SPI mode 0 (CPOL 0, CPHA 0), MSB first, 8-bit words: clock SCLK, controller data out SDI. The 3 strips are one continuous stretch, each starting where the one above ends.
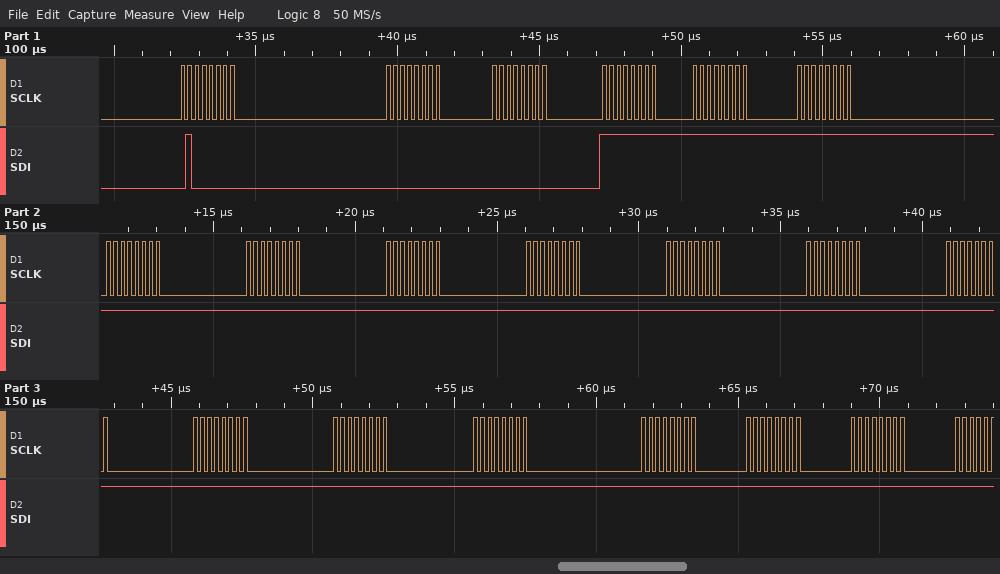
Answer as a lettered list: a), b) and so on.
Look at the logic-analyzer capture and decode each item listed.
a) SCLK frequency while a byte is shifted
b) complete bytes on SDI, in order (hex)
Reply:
a) 4 MHz
b) 40 00 00 FF FF FF FF FF FF FF FF FF FF FF FF FF FF FF FF
